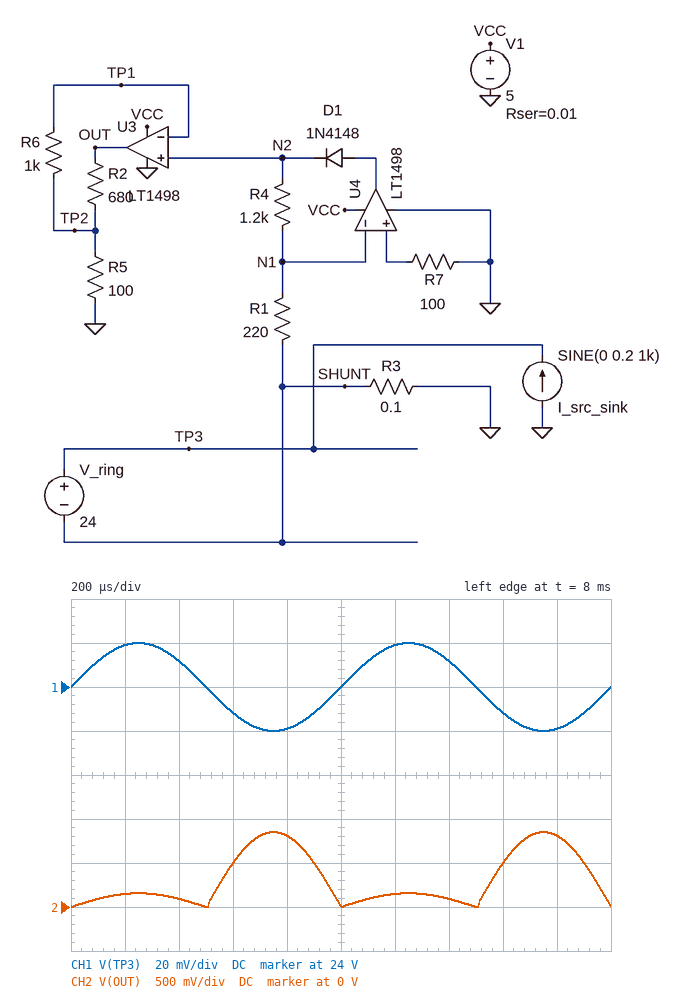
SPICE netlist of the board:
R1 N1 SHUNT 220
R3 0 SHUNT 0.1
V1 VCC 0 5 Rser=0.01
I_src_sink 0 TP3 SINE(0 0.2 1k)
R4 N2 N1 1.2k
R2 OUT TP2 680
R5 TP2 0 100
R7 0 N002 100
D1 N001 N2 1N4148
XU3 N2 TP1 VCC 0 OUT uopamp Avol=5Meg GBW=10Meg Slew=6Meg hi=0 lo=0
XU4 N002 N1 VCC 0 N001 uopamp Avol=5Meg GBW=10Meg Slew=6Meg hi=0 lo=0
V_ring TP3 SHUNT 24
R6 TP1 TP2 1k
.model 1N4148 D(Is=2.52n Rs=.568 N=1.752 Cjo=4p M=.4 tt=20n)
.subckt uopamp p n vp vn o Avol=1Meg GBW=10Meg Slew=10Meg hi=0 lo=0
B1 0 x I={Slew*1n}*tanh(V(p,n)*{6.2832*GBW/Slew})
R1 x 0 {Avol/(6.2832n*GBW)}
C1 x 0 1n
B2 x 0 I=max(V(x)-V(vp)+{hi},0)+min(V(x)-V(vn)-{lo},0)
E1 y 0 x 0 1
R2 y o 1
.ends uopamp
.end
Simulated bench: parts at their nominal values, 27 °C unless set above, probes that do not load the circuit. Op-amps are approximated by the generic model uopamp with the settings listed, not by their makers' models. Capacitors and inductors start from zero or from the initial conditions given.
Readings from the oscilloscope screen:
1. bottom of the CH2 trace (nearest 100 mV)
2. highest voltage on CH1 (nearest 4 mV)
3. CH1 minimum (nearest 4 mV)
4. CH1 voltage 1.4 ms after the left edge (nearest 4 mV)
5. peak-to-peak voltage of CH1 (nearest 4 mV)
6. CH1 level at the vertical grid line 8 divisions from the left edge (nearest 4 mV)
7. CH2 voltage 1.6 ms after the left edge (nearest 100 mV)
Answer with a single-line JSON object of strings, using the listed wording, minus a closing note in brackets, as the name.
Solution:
{"bottom of the CH2 trace": "0 V", "highest voltage on CH1": "24.020 V", "CH1 minimum": "23.980 V", "CH1 voltage 1.4 ms after the left edge": "24.012 V", "peak-to-peak voltage of CH1": "40 mV", "CH1 level at the vertical grid line 8 divisions from the left edge": "23.988 V", "CH2 voltage 1.6 ms after the left edge": "500 mV"}
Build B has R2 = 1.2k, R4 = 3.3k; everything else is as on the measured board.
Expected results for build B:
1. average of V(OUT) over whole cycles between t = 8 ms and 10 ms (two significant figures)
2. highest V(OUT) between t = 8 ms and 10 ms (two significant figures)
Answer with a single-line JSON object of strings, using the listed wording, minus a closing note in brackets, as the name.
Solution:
{"average of V(OUT) over whole cycles between t = 8 ms and 10 ms": "1.3 V", "highest V(OUT) between t = 8 ms and 10 ms": "3.9 V"}
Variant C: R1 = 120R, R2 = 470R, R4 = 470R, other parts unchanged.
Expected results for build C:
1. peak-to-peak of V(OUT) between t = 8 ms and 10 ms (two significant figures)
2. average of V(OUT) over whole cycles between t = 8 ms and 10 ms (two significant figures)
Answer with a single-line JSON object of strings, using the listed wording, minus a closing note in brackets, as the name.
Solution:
{"peak-to-peak of V(OUT) between t = 8 ms and 10 ms": "450 mV", "average of V(OUT) over whole cycles between t = 8 ms and 10 ms": "180 mV"}
